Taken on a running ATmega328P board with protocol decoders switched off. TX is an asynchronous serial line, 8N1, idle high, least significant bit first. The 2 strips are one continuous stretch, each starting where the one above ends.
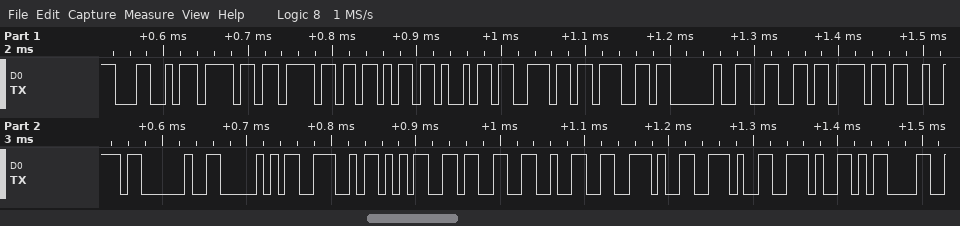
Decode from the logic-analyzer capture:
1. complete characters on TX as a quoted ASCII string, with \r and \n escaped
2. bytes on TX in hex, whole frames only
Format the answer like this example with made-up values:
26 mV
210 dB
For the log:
"Looking for PN532...\r"
4C 6F 6F 6B 69 6E 67 20 66 6F 72 20 50 4E 35 33 32 2E 2E 2E 0D
